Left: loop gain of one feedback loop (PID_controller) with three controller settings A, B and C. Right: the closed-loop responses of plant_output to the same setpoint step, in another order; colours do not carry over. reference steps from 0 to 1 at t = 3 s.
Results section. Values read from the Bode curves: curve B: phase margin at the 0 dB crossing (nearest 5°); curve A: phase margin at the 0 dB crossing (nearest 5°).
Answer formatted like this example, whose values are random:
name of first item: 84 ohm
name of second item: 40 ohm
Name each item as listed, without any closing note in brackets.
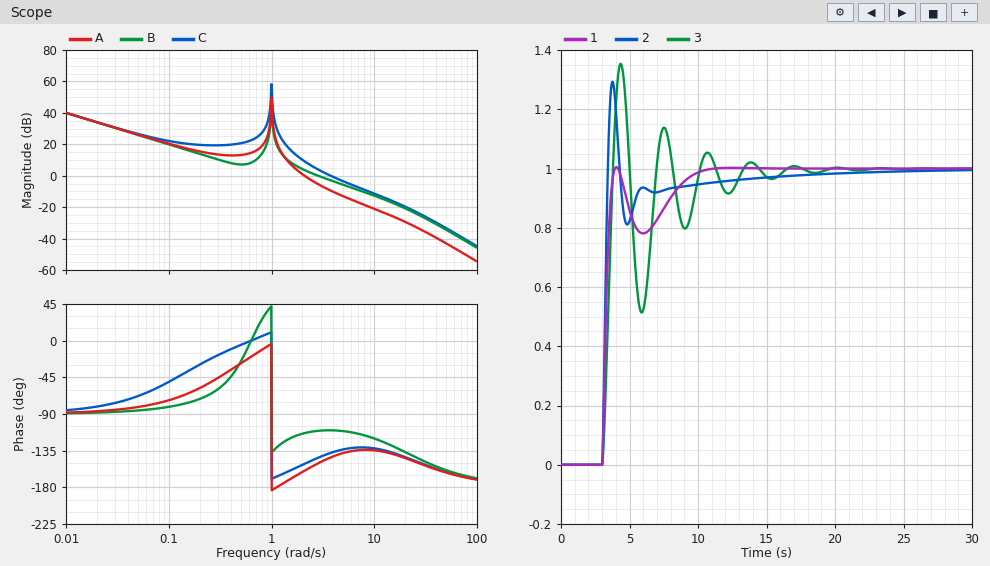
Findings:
curve B: phase margin at the 0 dB crossing: 70°
curve A: phase margin at the 0 dB crossing: 20°
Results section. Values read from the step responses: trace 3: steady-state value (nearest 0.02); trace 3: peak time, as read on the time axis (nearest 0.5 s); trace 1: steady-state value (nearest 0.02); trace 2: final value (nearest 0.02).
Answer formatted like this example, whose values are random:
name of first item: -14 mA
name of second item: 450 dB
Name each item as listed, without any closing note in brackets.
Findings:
trace 3: steady-state value: 1.00
trace 3: peak time, as read on the time axis: 4.5 s
trace 1: steady-state value: 1.00
trace 2: final value: 1.00
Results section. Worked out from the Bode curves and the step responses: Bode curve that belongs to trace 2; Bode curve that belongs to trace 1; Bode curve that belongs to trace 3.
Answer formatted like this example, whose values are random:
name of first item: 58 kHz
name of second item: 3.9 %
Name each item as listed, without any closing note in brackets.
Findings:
Bode curve that belongs to trace 2: C
Bode curve that belongs to trace 1: B
Bode curve that belongs to trace 3: A
